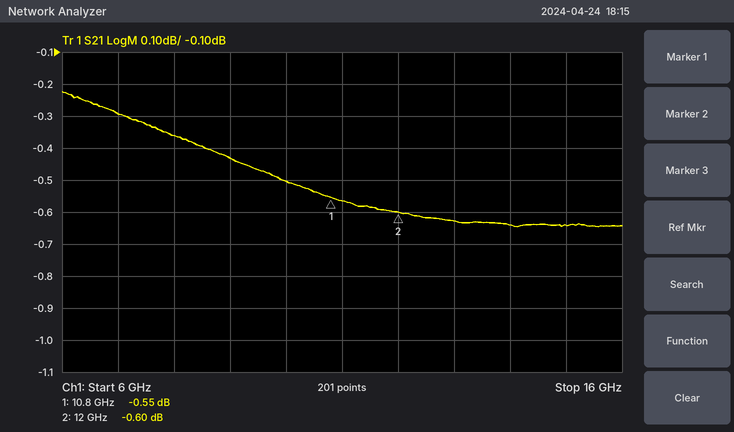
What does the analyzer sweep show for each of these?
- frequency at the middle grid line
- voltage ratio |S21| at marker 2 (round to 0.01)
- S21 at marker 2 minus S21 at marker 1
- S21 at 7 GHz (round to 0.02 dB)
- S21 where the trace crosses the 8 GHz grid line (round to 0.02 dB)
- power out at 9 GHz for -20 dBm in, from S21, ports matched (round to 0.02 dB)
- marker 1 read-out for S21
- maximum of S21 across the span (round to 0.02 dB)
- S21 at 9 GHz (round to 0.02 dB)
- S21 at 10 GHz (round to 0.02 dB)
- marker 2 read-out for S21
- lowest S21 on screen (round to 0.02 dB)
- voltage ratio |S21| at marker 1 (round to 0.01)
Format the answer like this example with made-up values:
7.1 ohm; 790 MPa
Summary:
11 GHz; 0.93; -0.05 dB; -0.30 dB; -0.36 dB; -20.44 dBm; -0.55 dB; -0.22 dB; -0.44 dB; -0.50 dB; -0.60 dB; -0.64 dB; 0.94
